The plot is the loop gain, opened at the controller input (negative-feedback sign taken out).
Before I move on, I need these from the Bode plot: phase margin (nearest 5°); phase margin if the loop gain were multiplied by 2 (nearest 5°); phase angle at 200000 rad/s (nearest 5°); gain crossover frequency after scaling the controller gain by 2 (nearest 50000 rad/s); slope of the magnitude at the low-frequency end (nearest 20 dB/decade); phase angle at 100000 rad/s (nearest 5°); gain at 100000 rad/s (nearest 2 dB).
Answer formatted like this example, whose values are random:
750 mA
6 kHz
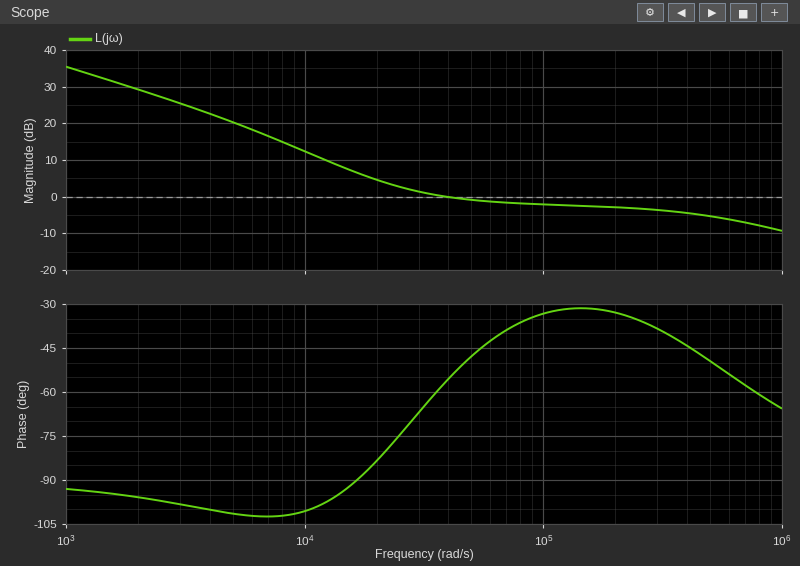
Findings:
125°
125°
-35°
600000 rad/s
-20 dB/decade
-35°
-2 dB
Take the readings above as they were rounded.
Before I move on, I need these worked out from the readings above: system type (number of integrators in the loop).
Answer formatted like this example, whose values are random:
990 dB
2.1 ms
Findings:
1
